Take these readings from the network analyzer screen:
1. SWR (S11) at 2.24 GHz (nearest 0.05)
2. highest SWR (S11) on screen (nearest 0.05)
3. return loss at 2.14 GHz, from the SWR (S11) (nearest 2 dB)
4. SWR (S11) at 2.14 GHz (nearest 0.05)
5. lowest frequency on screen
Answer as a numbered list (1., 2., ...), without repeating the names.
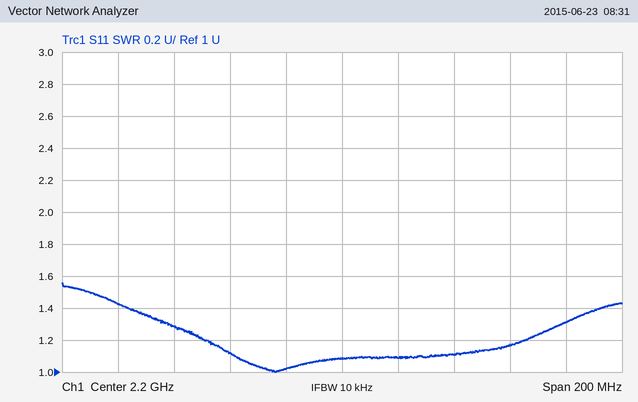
1. 1.10
2. 1.55
3. 18 dB
4. 1.30
5. 2.1 GHz
